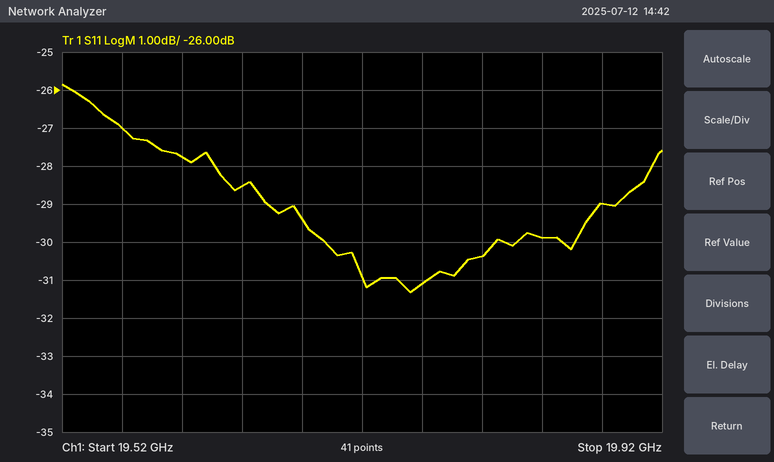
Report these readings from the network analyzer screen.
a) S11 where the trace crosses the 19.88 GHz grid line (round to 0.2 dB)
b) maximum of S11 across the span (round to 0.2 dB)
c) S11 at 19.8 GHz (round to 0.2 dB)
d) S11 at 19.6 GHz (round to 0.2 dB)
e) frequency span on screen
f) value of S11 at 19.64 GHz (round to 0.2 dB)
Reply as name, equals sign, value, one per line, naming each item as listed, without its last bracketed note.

S11 where the trace crosses the 19.88 GHz grid line = -29.0 dB
maximum of S11 across the span = -25.8 dB
S11 at 19.8 GHz = -30.4 dB
S11 at 19.6 GHz = -27.8 dB
frequency span on screen = 400 MHz
value of S11 at 19.64 GHz = -28.6 dB
